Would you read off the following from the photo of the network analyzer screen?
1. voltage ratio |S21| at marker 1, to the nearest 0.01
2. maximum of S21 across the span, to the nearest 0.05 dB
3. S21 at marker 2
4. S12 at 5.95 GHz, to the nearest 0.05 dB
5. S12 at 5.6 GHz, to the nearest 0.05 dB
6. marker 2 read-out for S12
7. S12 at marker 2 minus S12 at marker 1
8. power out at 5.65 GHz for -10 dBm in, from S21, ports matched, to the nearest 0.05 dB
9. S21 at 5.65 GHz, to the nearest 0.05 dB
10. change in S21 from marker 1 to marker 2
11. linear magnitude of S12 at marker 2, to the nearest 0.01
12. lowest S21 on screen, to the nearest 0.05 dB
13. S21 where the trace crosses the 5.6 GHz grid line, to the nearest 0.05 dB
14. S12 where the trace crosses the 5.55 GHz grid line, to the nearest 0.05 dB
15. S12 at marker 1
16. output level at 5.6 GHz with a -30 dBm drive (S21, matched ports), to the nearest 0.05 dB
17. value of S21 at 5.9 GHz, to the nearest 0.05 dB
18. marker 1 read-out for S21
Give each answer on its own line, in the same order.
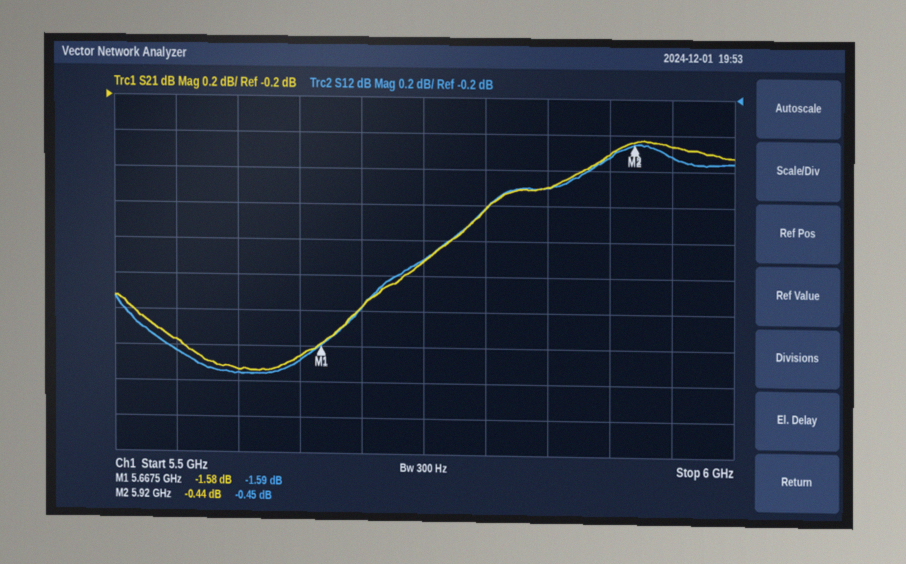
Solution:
0.83
-0.45 dB
-0.44 dB
-0.50 dB
-1.75 dB
-0.45 dB
1.14 dB
-11.65 dBm
-1.65 dB
1.14 dB
0.95
-1.75 dB
-1.75 dB
-1.65 dB
-1.59 dB
-31.75 dBm
-0.50 dB
-1.58 dB
